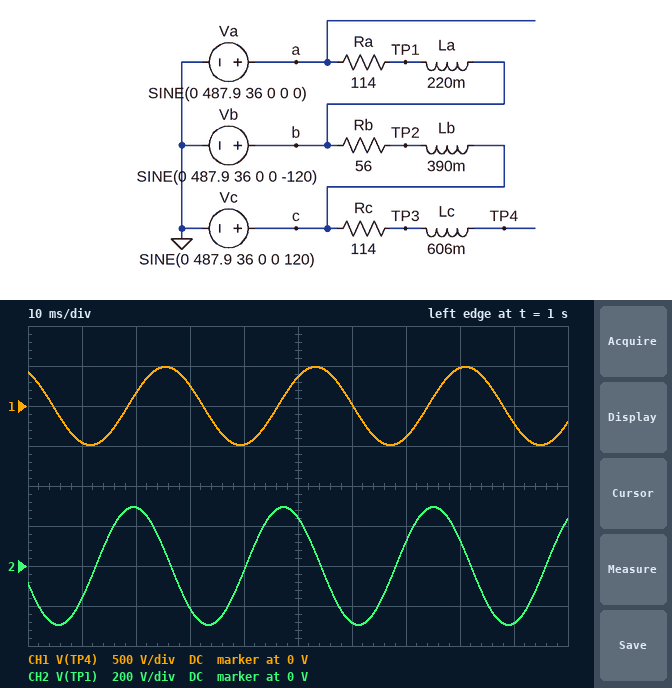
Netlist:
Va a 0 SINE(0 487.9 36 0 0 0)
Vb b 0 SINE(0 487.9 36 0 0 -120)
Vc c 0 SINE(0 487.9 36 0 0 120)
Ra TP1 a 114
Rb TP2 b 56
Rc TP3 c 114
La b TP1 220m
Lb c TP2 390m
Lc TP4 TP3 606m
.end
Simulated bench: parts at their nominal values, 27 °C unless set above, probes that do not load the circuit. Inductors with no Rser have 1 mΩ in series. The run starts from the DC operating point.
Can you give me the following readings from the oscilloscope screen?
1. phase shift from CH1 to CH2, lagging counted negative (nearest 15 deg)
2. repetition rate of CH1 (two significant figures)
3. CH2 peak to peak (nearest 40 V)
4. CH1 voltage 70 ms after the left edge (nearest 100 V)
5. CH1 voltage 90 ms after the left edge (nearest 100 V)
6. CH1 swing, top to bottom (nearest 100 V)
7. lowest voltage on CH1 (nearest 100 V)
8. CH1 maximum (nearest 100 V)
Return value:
75 deg
36 Hz
600 V
-400 V
-200 V
1.0 kV
-500 V
500 V
